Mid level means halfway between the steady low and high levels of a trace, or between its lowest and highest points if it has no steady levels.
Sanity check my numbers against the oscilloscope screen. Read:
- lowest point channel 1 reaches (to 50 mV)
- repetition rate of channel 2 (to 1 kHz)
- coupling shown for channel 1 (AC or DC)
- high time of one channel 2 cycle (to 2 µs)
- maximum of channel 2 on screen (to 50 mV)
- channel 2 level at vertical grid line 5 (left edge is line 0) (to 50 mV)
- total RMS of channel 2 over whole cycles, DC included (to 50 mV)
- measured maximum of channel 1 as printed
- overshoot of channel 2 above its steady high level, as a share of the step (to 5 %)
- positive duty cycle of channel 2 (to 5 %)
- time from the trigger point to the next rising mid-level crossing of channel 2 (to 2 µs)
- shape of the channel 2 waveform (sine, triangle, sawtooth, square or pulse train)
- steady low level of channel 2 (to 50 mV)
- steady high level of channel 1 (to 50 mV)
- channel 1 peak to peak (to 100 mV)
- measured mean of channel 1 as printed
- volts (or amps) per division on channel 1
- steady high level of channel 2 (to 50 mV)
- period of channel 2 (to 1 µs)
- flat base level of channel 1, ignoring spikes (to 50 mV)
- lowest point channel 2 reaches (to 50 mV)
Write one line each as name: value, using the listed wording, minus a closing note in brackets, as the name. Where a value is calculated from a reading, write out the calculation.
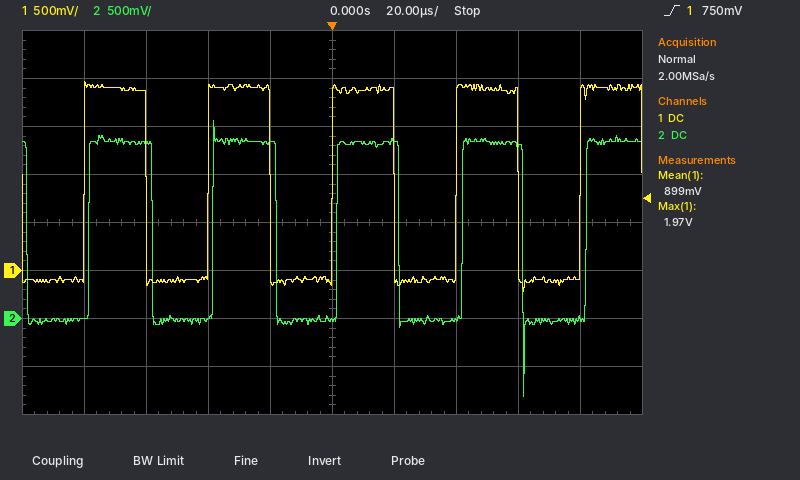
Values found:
lowest point channel 1 reaches: -200 mV
repetition rate of channel 2: 1 / 40 µs ≈ 25 kHz
coupling shown for channel 1: DC
high time of one channel 2 cycle: 20 µs
maximum of channel 2 on screen: 2.05 V
channel 2 level at vertical grid line 5 (left edge is line 0): 0 mV
total RMS of channel 2 over whole cycles, DC included: √(0.5 × (1.85 V)² + 0.5 × (0 mV)²) ≈ 1.31 V, so 1.30 V to the nearest 50 mV
measured maximum of channel 1 as printed: 1.97 V
overshoot of channel 2 above its steady high level, as a share of the step: 10 %
positive duty cycle of channel 2: 20 µs / 40 µs ≈ 50 %
time from the trigger point to the next rising mid-level crossing of channel 2: 2 µs
shape of the channel 2 waveform: square
steady low level of channel 2: 0 mV
steady high level of channel 1: 1.90 V
channel 1 peak to peak: 2.20 V
measured mean of channel 1 as printed: 899 mV
volts (or amps) per division on channel 1: 500 mV
steady high level of channel 2: 1.85 V
period of channel 2: 40 µs
flat base level of channel 1, ignoring spikes: -100 mV
lowest point channel 2 reaches: -800 mV
